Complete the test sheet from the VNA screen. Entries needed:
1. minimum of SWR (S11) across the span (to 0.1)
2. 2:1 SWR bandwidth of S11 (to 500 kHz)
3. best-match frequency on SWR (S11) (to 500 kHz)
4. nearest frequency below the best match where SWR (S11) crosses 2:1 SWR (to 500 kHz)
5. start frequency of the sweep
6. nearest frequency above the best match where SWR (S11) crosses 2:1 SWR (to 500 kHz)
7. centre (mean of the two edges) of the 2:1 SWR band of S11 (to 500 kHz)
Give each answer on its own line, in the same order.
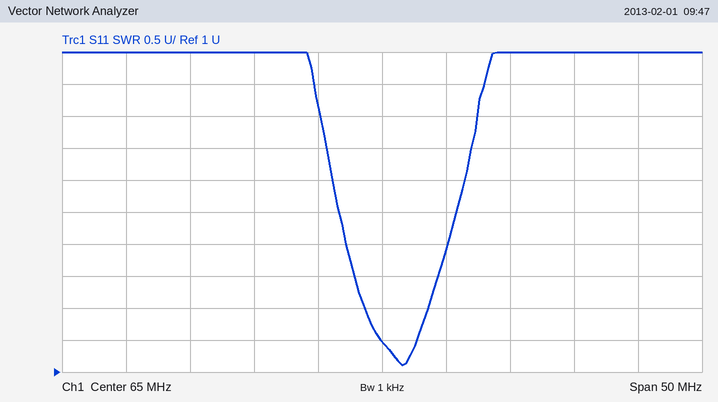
1.1
5.0 MHz
66.5 MHz
63.5 MHz
40 MHz
68.5 MHz
66.0 MHz
